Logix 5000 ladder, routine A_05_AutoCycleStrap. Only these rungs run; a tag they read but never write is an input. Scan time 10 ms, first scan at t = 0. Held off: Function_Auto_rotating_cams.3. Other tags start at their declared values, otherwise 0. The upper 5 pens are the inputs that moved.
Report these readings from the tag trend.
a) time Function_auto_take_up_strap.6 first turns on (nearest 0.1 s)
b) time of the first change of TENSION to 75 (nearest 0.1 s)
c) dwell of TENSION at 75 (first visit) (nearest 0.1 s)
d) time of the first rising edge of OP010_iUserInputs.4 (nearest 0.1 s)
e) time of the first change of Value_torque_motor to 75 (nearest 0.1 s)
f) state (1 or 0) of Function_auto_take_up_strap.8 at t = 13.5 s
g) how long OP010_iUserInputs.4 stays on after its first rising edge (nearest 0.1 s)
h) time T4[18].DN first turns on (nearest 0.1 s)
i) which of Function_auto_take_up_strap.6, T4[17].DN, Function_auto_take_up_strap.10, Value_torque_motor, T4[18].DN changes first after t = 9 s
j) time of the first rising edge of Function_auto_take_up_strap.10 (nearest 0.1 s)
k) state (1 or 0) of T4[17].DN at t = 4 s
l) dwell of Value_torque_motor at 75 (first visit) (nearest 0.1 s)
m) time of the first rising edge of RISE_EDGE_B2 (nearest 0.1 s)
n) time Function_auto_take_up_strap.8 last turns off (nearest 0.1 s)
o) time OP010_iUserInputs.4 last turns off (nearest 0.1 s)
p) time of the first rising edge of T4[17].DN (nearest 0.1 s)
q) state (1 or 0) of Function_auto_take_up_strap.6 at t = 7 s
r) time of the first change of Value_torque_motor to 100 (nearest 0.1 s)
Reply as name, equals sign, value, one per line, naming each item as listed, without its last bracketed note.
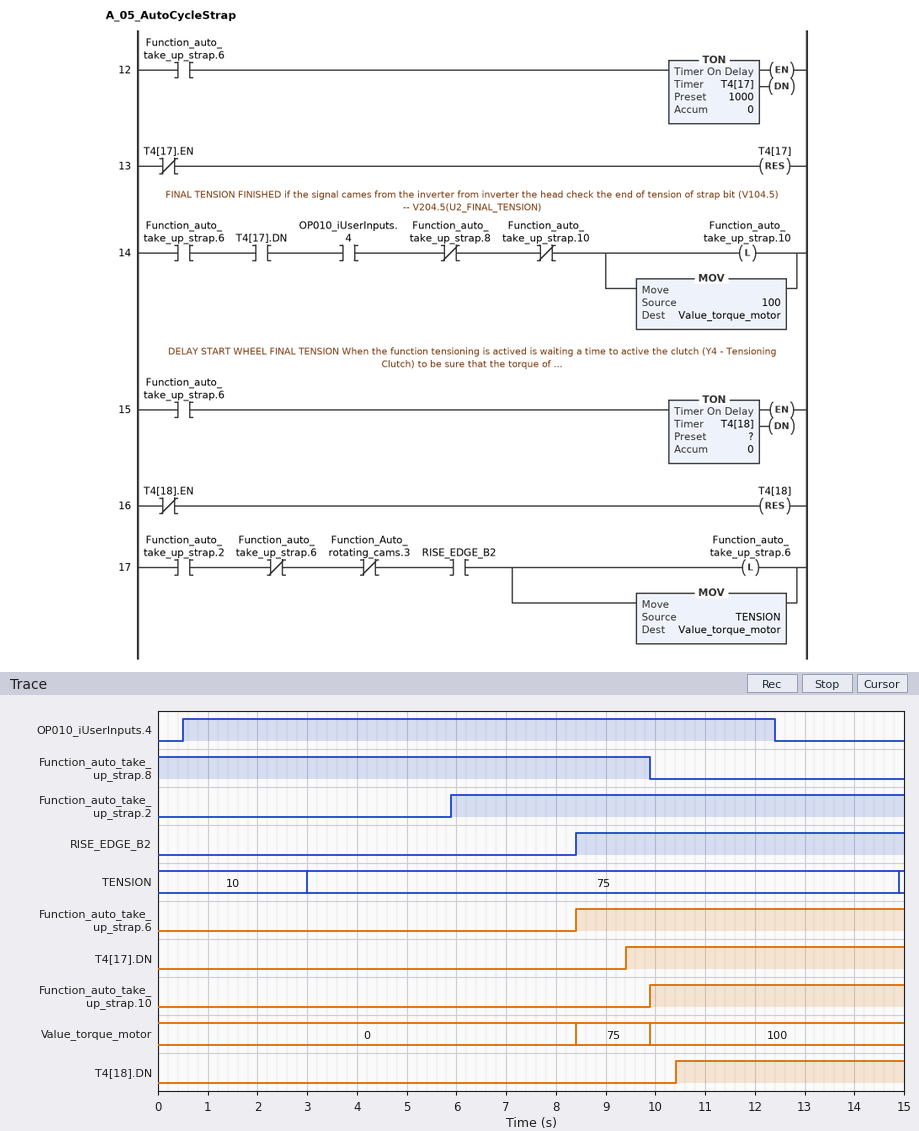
time Function_auto_take_up_strap.6 first turns on = 8.4 s
time of the first change of TENSION to 75 = 3.0 s
dwell of TENSION at 75 (first visit) = 11.9 s
time of the first rising edge of OP010_iUserInputs.4 = 0.5 s
time of the first change of Value_torque_motor to 75 = 8.4 s
state (1 or 0) of Function_auto_take_up_strap.8 at t = 13.5 s = 0
how long OP010_iUserInputs.4 stays on after its first rising edge = 11.9 s
time T4[18].DN first turns on = 10.4 s
which of Function_auto_take_up_strap.6, T4[17].DN, Function_auto_take_up_strap.10, Value_torque_motor, T4[18].DN changes first after t = 9 s = T4[17].DN
time of the first rising edge of Function_auto_take_up_strap.10 = 9.9 s
state (1 or 0) of T4[17].DN at t = 4 s = 0
dwell of Value_torque_motor at 75 (first visit) = 1.5 s
time of the first rising edge of RISE_EDGE_B2 = 8.4 s
time Function_auto_take_up_strap.8 last turns off = 9.9 s
time OP010_iUserInputs.4 last turns off = 12.4 s
time of the first rising edge of T4[17].DN = 9.4 s
state (1 or 0) of Function_auto_take_up_strap.6 at t = 7 s = 0
time of the first change of Value_torque_motor to 100 = 9.9 s
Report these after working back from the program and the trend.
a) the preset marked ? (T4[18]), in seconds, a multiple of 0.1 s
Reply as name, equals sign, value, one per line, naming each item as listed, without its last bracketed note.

the preset marked ? (T4[18]), in seconds, a multiple of 0.1 s = 2.0 s
